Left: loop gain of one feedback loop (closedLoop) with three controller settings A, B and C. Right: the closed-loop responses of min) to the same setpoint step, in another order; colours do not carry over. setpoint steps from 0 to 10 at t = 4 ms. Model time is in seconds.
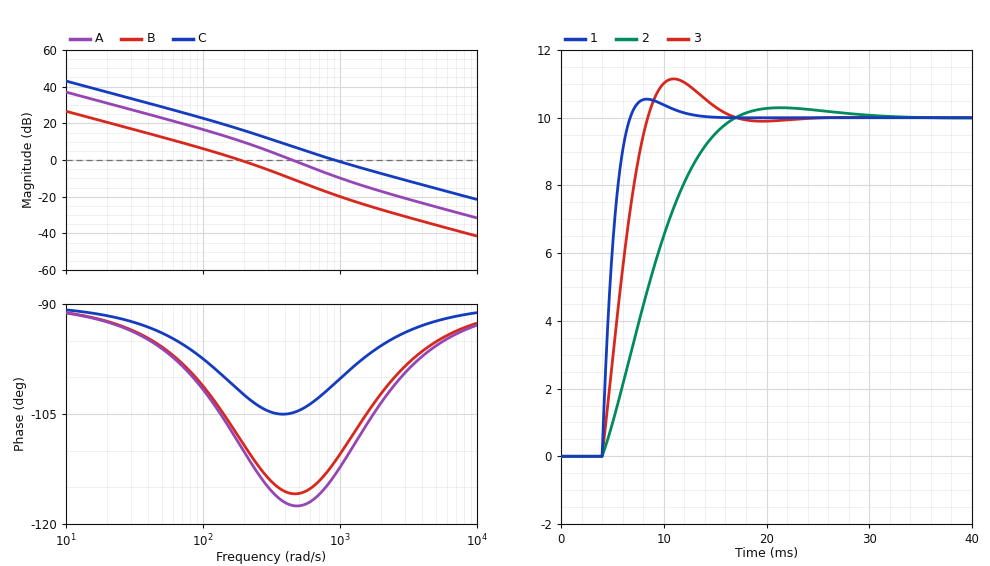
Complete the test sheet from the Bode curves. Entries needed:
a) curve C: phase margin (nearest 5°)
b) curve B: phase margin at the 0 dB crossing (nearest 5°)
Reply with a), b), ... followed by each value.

a) 80°
b) 70°
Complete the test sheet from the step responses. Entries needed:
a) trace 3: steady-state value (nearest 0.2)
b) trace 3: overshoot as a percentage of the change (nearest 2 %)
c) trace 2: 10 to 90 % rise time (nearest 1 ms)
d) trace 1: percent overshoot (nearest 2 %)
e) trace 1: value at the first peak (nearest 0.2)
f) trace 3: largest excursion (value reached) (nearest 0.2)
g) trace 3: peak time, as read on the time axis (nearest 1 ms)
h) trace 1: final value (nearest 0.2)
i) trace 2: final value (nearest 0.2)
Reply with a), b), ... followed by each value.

a) 10.0
b) 12 %
c) 9 ms
d) 6 %
e) 10.6
f) 11.2
g) 11 ms
h) 10.0
i) 10.0
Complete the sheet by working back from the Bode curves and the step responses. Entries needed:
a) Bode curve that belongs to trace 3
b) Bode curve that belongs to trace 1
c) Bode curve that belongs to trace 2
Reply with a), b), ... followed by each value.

a) A
b) C
c) B
